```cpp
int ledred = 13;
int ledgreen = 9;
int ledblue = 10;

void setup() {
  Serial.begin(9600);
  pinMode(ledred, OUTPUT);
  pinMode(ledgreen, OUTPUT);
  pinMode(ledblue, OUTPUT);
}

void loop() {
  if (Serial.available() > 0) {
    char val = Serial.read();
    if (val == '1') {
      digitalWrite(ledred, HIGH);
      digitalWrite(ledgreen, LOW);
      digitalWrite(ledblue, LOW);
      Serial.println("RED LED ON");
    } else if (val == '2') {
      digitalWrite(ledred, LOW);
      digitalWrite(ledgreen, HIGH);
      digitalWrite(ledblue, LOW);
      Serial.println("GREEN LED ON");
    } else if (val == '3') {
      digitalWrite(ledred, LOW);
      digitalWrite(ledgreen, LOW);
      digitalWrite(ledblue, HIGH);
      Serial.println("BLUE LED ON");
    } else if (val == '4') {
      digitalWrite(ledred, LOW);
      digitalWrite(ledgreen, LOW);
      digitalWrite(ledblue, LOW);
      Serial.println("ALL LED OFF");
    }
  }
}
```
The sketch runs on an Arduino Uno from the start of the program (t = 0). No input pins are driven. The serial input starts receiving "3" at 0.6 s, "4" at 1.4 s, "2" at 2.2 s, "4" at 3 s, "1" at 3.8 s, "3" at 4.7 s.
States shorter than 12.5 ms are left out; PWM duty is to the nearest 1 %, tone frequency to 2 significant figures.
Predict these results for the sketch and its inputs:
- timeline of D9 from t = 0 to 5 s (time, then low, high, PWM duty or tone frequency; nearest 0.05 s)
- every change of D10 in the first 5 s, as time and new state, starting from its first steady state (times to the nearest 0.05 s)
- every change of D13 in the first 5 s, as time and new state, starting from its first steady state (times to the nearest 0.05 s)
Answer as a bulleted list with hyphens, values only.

- 0 s low; 2.2 s high; 3 s low
- 0 s low; 0.6 s high; 1.4 s low; 4.7 s high
- 0 s low; 3.8 s high; 4.7 s low
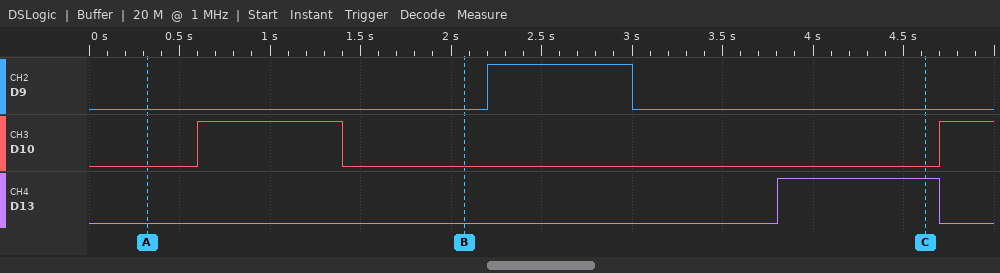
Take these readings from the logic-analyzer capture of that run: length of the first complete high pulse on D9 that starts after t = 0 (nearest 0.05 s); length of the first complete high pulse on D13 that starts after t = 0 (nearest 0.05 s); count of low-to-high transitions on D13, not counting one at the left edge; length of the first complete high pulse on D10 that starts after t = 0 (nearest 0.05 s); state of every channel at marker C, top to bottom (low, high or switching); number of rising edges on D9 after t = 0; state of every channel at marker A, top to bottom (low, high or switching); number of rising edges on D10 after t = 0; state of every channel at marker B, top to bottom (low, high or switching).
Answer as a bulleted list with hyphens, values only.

- 0.80 s
- 0.90 s
- 1
- 0.80 s
- D9 low, D10 low, D13 high
- 1
- D9 low, D10 low, D13 low
- 2
- D9 low, D10 low, D13 low
